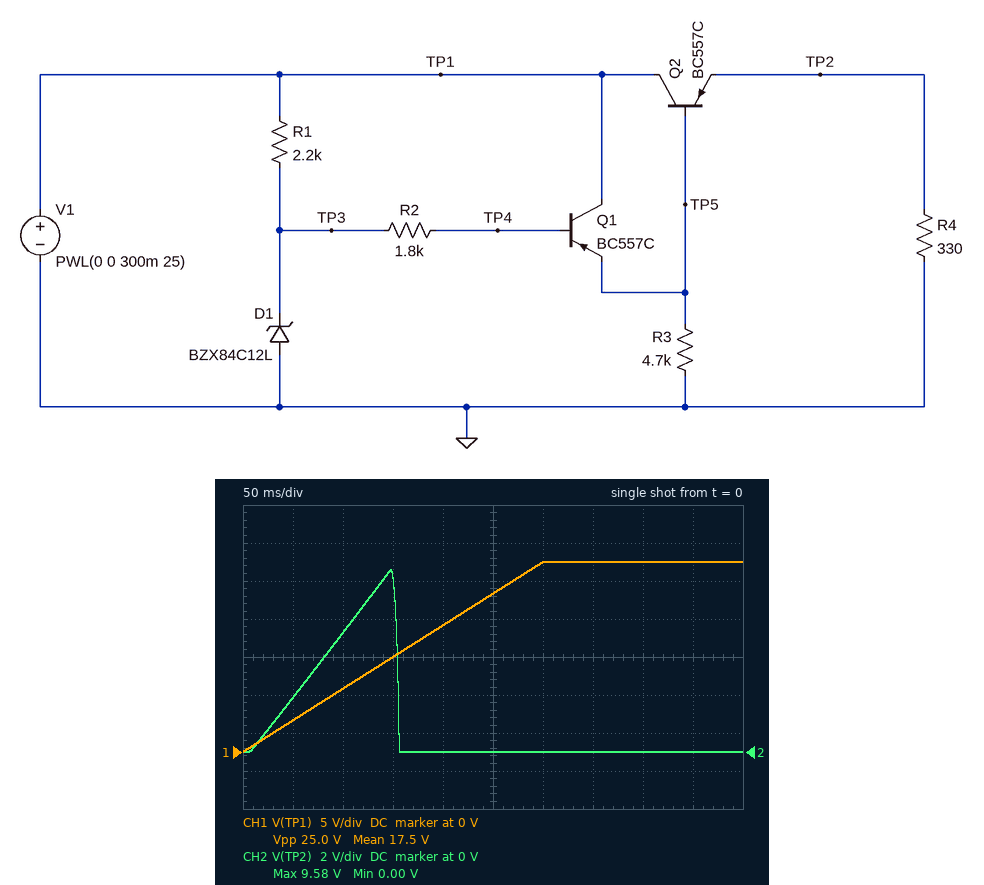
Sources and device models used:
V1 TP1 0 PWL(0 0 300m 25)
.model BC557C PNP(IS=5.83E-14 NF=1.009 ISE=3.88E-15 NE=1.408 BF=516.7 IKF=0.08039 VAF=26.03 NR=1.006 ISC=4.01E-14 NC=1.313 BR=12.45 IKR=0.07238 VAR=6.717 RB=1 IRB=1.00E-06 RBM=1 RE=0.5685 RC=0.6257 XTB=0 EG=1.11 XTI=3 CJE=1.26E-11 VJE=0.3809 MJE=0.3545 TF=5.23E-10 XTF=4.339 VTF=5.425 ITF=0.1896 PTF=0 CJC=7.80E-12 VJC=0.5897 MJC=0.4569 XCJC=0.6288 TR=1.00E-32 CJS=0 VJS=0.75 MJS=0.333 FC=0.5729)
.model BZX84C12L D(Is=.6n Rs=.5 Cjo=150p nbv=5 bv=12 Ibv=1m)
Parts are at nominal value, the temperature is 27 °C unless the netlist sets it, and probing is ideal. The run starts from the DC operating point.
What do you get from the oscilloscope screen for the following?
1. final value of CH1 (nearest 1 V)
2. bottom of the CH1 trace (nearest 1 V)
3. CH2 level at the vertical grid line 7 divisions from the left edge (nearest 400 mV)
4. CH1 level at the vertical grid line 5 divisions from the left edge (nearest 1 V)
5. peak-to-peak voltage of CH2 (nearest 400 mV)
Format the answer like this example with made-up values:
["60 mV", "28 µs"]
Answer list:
["25 V", "0 V", "0 V", "21 V", "9.6 V"]
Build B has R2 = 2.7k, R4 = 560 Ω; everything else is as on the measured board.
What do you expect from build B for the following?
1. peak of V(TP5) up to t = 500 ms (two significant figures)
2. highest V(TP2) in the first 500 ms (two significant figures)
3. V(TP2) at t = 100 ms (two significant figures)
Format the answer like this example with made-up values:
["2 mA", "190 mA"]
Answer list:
["25 V", "12 V", "8.1 V"]
